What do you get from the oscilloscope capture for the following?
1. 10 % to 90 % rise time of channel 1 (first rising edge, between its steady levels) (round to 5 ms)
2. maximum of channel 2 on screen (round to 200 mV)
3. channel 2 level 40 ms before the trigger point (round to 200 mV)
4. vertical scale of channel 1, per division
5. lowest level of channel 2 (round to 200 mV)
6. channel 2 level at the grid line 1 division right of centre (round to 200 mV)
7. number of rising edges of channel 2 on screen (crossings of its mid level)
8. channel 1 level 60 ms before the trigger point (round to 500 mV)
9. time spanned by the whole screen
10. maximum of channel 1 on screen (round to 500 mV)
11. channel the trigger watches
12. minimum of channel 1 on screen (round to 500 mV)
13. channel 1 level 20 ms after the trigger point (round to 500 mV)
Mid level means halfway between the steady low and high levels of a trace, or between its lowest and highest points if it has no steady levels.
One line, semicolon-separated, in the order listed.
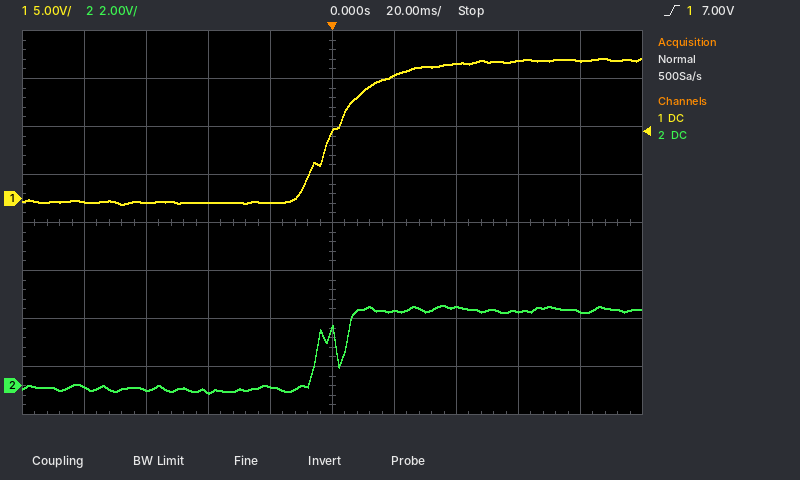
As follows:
30 ms; 3.4 V; -200 mV; 5 V; -400 mV; 3.2 V; 2; -500 mV; 200 ms; 14.5 V; channel 1; -500 mV; 13.0 V
